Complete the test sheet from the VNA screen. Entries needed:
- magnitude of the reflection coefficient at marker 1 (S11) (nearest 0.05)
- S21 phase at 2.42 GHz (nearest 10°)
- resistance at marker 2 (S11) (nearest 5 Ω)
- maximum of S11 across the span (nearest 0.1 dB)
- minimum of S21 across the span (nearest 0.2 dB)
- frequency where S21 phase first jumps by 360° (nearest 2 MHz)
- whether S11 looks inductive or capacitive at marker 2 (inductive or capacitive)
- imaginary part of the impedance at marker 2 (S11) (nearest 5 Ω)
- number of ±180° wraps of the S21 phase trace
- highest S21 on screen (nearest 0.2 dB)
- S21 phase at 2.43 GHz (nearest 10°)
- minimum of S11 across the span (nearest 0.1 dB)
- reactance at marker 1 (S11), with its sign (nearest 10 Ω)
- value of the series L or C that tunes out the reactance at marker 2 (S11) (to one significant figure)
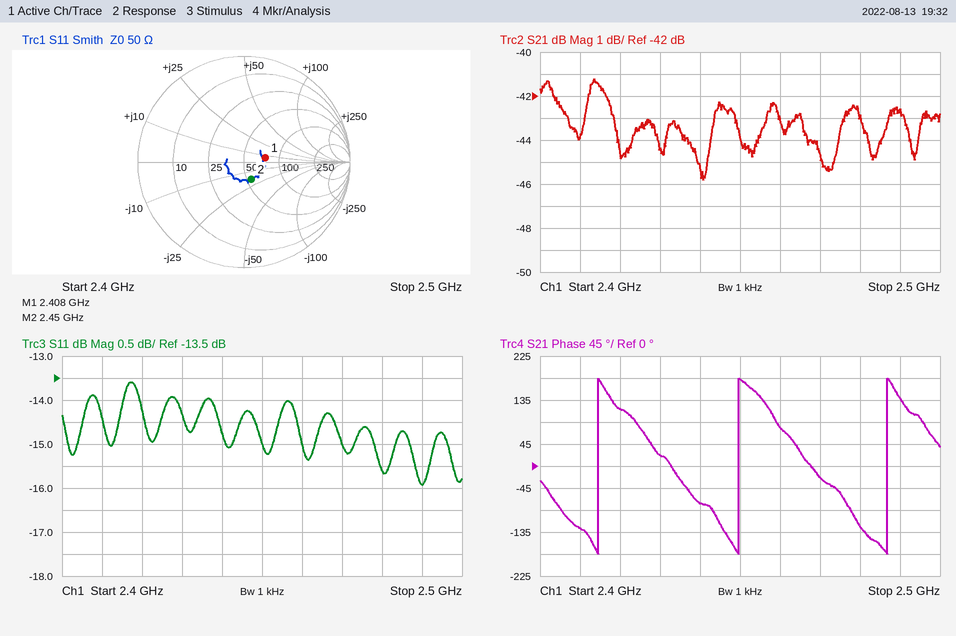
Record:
0.20
120°
55 Ω
-13.6 dB
-45.8 dB
2.414 GHz
capacitive
-20 Ω
3
-41.2 dB
20°
-15.9 dB
+10 Ω
1 nH
